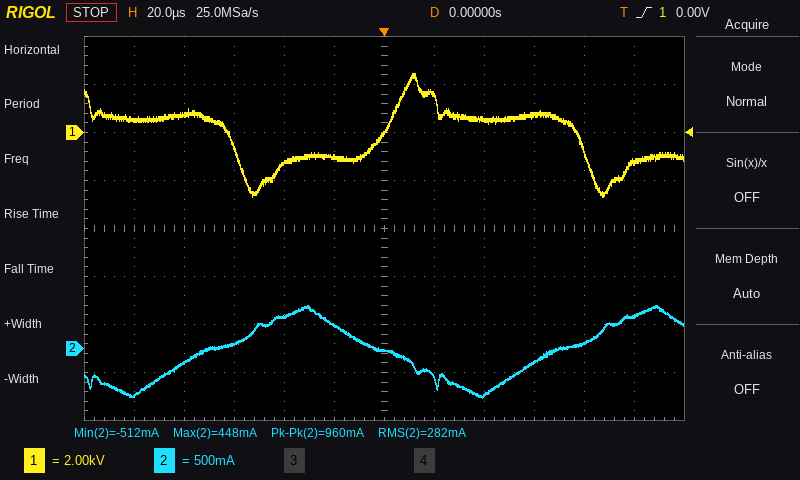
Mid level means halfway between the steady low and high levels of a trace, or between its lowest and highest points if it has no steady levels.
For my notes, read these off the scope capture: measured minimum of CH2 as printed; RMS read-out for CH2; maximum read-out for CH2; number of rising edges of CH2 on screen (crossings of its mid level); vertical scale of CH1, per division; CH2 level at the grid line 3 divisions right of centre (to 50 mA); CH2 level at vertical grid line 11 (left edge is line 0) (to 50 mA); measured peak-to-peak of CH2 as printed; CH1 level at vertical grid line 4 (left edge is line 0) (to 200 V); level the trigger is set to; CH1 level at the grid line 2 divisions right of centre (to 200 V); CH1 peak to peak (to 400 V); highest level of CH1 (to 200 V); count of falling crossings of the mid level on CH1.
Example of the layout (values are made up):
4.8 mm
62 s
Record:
-512 mA
282 mA
448 mA
2
2 kV
-150 mA
350 mA
960 mA
-1.2 kV
0.00 V
600 V
5.2 kV
2.4 kV
2
